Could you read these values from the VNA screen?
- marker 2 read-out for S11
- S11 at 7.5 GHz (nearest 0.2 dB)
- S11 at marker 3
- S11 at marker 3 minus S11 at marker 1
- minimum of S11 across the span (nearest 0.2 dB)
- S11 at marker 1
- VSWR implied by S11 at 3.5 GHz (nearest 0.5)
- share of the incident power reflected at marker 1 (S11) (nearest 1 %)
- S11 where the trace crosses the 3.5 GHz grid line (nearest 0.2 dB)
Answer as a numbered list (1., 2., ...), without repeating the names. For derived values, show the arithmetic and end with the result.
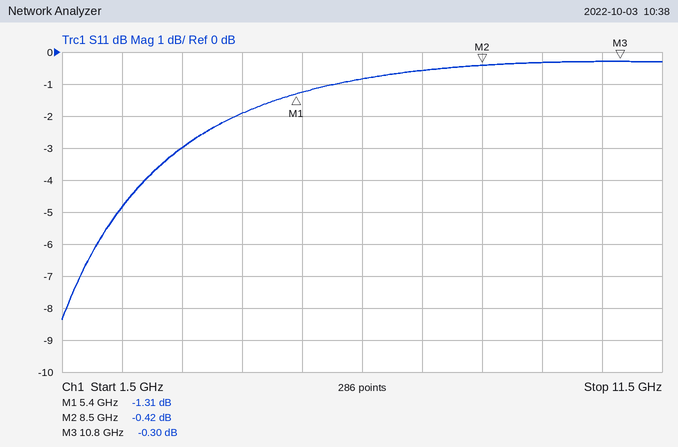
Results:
1. -0.42 dB
2. -0.6 dB
3. -0.30 dB
4. -0.3 − (-1.31) = 1.01 dB
5. -8.4 dB
6. -1.31 dB
7. |Γ| = 10^(-3/20) = 0.7079; VSWR = (1 + 0.7079)/(1 − 0.7079) ≈ 5.85, so 6.0 to the nearest 0.5
8. 10^(-1.31/10) ≈ 74 %
9. -3.0 dB
